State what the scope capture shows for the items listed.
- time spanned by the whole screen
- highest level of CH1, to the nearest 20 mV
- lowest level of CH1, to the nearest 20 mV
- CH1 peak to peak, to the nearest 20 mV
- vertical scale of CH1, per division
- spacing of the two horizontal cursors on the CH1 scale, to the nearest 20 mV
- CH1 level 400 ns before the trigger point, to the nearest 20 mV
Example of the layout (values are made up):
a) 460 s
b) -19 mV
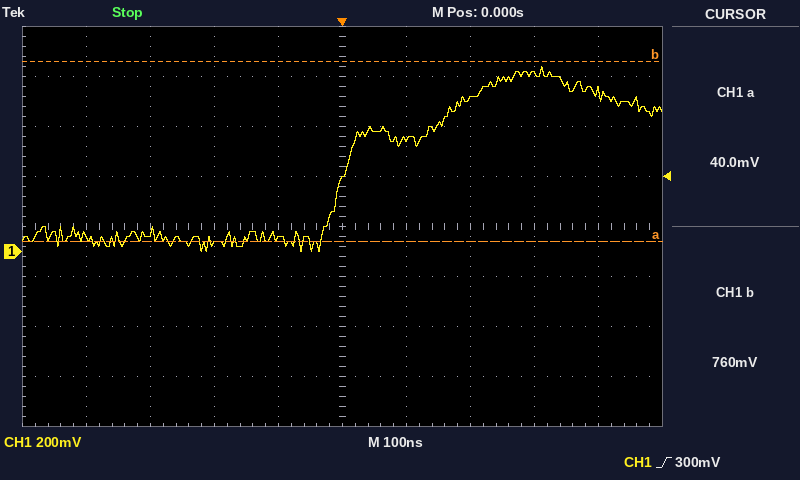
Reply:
a) 1 µs
b) 740 mV
c) 0 mV
d) 740 mV
e) 200 mV
f) 720 mV
g) 60 mV
